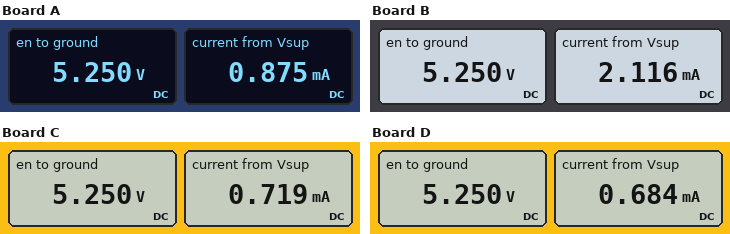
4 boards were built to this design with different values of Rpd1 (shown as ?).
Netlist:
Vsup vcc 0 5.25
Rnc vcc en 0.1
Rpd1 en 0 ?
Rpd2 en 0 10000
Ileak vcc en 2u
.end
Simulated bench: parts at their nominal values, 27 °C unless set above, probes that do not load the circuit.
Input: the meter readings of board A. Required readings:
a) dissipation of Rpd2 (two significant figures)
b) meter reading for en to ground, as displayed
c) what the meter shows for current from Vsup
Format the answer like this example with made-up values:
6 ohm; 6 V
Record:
2.8 mW; 5.250 V; 0.875 mA
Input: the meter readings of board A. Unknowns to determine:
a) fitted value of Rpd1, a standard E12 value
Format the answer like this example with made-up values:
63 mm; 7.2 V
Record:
15 kΩ
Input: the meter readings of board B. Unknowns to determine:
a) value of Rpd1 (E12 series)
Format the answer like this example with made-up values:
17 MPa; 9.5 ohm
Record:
3.3 kΩ
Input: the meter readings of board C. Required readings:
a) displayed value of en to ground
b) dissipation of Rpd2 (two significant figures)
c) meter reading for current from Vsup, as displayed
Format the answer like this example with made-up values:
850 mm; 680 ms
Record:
5.250 V; 2.8 mW; 0.719 mA
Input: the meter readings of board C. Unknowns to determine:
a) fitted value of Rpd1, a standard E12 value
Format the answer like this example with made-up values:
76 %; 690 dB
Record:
27 kΩ
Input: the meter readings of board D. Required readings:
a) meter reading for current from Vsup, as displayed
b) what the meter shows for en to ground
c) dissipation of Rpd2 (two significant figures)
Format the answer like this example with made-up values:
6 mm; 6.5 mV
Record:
0.684 mA; 5.250 V; 2.8 mW
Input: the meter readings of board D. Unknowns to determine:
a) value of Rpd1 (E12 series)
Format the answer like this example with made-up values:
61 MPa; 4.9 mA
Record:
33 kΩ
